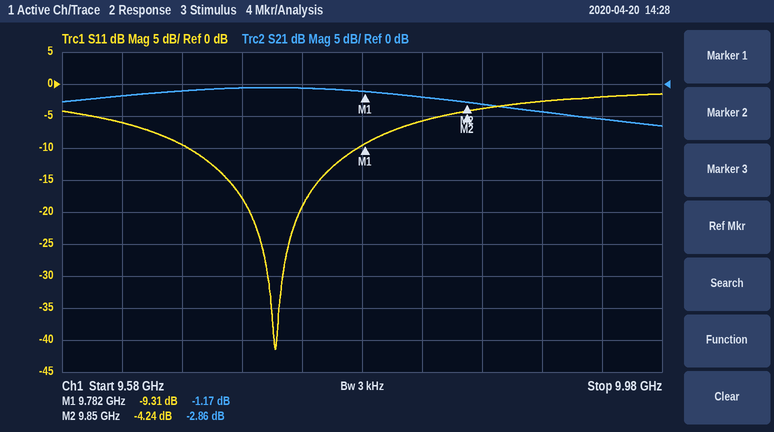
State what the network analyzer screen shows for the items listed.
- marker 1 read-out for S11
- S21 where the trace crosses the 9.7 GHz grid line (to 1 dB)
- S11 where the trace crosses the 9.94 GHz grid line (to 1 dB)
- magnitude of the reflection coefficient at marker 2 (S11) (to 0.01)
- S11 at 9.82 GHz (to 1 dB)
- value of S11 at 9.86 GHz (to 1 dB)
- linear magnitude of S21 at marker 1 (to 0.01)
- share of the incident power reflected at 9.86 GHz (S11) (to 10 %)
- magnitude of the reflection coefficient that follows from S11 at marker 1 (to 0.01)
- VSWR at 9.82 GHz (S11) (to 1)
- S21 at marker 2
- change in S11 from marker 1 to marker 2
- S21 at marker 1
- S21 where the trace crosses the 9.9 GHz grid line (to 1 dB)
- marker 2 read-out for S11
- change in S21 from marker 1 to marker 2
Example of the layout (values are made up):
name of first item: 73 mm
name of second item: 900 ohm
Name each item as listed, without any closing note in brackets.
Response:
marker 1 read-out for S11: -9.31 dB
S21 where the trace crosses the 9.7 GHz grid line: -1 dB
S11 where the trace crosses the 9.94 GHz grid line: -2 dB
magnitude of the reflection coefficient at marker 2 (S11): 0.61
S11 at 9.82 GHz: -6 dB
value of S11 at 9.86 GHz: -4 dB
linear magnitude of S21 at marker 1: 0.87
share of the incident power reflected at 9.86 GHz (S11): 40 %
magnitude of the reflection coefficient that follows from S11 at marker 1: 0.34
VSWR at 9.82 GHz (S11): 3
S21 at marker 2: -2.86 dB
change in S11 from marker 1 to marker 2: 5.07 dB
S21 at marker 1: -1.17 dB
S21 where the trace crosses the 9.9 GHz grid line: -4 dB
marker 2 read-out for S11: -4.24 dB
change in S21 from marker 1 to marker 2: -1.69 dB
